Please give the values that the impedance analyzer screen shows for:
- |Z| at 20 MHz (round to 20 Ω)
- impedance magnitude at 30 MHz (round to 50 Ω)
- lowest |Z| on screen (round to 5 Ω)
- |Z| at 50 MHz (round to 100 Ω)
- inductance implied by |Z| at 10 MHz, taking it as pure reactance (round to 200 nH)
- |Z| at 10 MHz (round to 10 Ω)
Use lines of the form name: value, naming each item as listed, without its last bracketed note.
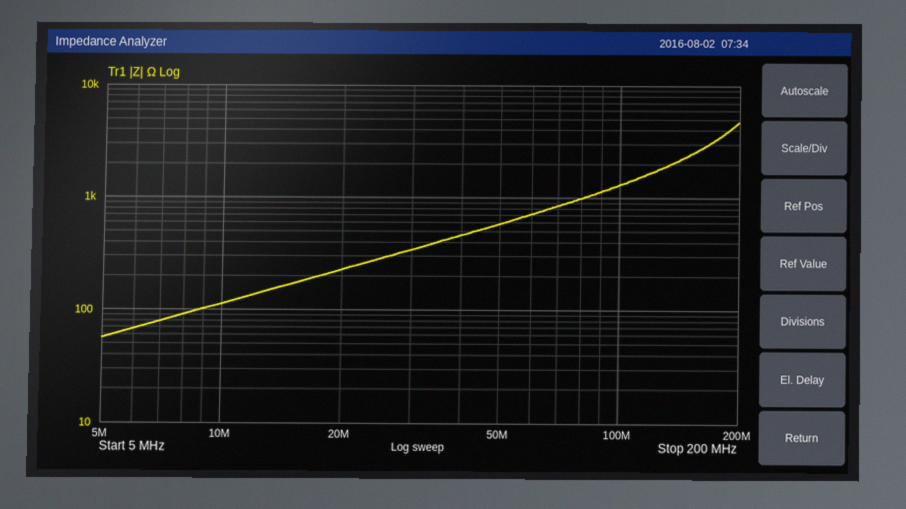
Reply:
|Z| at 20 MHz: 220 Ω
impedance magnitude at 30 MHz: 350 Ω
lowest |Z| on screen: 55 Ω
|Z| at 50 MHz: 600 Ω
inductance implied by |Z| at 10 MHz, taking it as pure reactance: 1.8 µH
|Z| at 10 MHz: 110 Ω
